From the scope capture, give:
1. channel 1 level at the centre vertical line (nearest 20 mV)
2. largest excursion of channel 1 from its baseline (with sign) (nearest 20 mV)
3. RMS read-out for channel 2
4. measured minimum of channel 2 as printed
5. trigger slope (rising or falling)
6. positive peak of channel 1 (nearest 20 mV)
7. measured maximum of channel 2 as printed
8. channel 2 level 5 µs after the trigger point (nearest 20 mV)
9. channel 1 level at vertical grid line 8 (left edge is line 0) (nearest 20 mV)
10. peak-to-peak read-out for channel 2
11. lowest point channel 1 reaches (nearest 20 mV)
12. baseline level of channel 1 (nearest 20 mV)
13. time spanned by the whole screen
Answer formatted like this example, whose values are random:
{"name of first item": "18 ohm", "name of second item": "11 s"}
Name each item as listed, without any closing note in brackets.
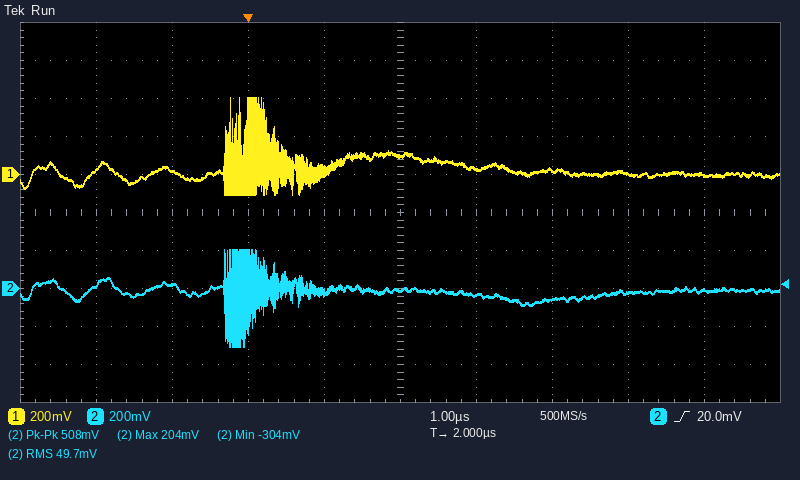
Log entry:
{"channel 1 level at the centre vertical line": "100 mV", "largest excursion of channel 1 from its baseline (with sign)": "+400 mV", "RMS read-out for channel 2": "49.7 mV", "measured minimum of channel 2 as printed": "-304 mV", "trigger slope": "rising", "positive peak of channel 1": "400 mV", "measured maximum of channel 2 as printed": "204 mV", "channel 2 level 5 µs after the trigger point": "-20 mV", "channel 1 level at vertical grid line 8 (left edge is line 0)": "0 mV", "peak-to-peak read-out for channel 2": "508 mV", "lowest point channel 1 reaches": "-100 mV", "baseline level of channel 1": "0 mV", "time spanned by the whole screen": "10 µs"}
